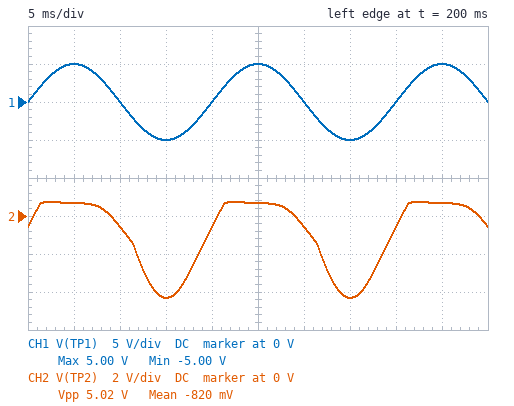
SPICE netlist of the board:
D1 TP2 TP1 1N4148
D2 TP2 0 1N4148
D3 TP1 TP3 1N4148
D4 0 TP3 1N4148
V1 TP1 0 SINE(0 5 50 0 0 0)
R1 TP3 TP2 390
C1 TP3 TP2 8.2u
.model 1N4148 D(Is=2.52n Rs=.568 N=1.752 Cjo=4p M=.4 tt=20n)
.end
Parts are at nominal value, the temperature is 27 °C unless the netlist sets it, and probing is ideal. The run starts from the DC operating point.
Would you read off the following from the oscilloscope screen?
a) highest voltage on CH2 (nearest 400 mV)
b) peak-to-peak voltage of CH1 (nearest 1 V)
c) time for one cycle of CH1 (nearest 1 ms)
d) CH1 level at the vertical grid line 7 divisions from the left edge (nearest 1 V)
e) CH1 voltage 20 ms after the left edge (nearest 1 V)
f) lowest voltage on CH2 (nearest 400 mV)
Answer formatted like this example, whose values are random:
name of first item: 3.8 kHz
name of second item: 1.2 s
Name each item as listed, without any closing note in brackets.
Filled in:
highest voltage on CH2: 800 mV
peak-to-peak voltage of CH1: 10 V
time for one cycle of CH1: 20 ms
CH1 level at the vertical grid line 7 divisions from the left edge: -5 V
CH1 voltage 20 ms after the left edge: 0 V
lowest voltage on CH2: -4.4 V
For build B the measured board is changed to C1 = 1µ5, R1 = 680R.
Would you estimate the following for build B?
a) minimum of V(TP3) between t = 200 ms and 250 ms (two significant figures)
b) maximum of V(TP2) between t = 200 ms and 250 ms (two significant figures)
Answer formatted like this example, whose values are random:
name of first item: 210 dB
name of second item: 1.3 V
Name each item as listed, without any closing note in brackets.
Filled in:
minimum of V(TP3) between t = 200 ms and 250 ms: -670 mV
maximum of V(TP2) between t = 200 ms and 250 ms: 670 mV
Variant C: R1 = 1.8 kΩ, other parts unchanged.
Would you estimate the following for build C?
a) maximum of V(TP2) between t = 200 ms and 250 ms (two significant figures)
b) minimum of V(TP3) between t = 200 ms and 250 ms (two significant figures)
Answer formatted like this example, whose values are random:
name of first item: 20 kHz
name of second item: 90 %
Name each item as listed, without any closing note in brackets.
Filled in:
maximum of V(TP2) between t = 200 ms and 250 ms: 690 mV
minimum of V(TP3) between t = 200 ms and 250 ms: -690 mV
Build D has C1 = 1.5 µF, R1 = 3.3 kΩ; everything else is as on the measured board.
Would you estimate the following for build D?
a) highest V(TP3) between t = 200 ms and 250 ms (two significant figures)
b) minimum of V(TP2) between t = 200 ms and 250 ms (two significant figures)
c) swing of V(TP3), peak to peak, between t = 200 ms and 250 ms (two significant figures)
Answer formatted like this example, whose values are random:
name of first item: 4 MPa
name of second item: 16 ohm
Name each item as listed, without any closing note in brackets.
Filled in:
highest V(TP3) between t = 200 ms and 250 ms: 4.4 V
minimum of V(TP2) between t = 200 ms and 250 ms: -4.4 V
swing of V(TP3), peak to peak, between t = 200 ms and 250 ms: 5.0 V
